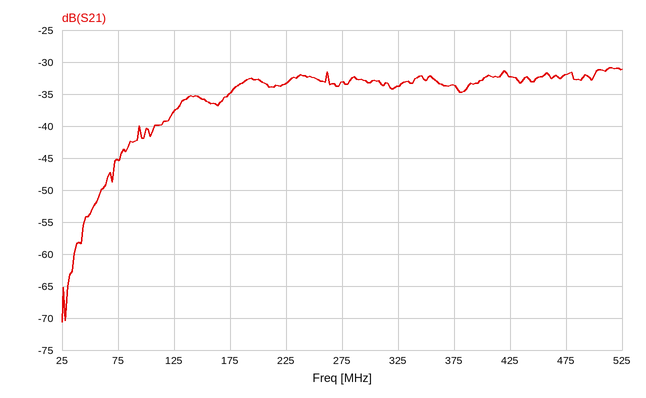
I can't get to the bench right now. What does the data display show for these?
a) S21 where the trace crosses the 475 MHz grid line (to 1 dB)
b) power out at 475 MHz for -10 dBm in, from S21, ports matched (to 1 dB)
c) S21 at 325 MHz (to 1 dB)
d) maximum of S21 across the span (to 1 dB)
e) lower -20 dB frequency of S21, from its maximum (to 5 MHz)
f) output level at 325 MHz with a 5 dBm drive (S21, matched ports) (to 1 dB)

-32 dB
-42 dBm
-34 dB
-31 dB
60 MHz
-29 dBm
